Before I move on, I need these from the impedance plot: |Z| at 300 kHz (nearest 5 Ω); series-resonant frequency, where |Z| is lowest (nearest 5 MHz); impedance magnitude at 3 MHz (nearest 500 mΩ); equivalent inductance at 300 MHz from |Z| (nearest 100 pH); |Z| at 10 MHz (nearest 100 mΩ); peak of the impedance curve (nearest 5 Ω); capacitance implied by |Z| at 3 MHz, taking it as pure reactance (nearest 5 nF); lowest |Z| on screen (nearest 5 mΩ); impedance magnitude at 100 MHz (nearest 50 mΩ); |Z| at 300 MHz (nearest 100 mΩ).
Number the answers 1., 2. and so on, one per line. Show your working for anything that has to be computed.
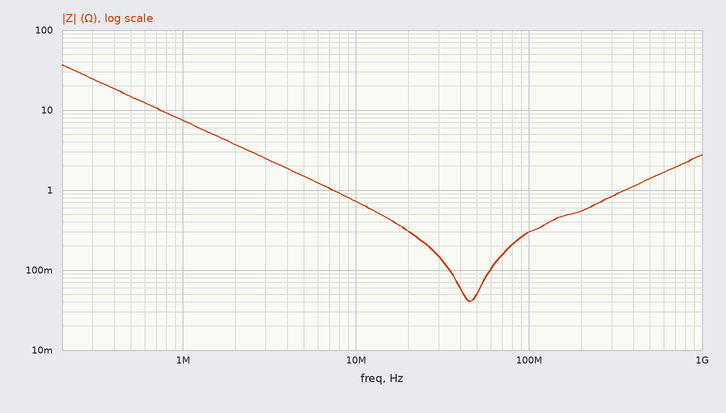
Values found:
1. 25 Ω
2. 45 MHz
3. 2.5 Ω
4. L = 800 mΩ/(2π × 300 MHz) ≈ 424 pH, so 400 pH to the nearest 100 pH
5. 700 mΩ
6. 35 Ω
7. C = 1/(2π × 3 MHz × 2.5 Ω) ≈ 21.2 nF, so 20 nF to the nearest 5 nF
8. 40 mΩ
9. 300 mΩ
10. 800 mΩ
